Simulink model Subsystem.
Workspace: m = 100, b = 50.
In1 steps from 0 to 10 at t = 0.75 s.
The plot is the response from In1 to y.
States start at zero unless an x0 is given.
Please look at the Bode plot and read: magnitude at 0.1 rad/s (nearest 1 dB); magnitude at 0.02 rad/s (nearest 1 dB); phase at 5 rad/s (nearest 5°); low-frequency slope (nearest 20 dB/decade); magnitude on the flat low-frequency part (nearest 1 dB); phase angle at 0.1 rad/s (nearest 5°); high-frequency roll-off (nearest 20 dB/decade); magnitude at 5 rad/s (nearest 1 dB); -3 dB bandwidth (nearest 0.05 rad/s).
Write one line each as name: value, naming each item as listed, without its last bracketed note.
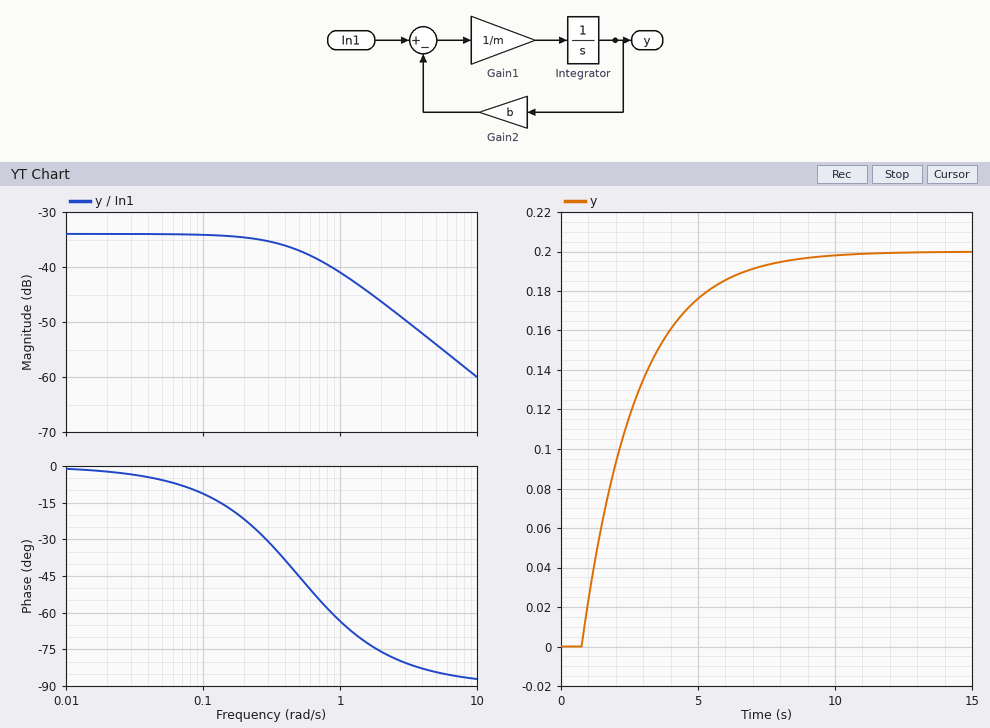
magnitude at 0.1 rad/s: -34 dB
magnitude at 0.02 rad/s: -34 dB
phase at 5 rad/s: -85°
low-frequency slope: 0 dB/decade
magnitude on the flat low-frequency part: -34 dB
phase angle at 0.1 rad/s: -10°
high-frequency roll-off: -20 dB/decade
magnitude at 5 rad/s: -54 dB
-3 dB bandwidth: 0.50 rad/s
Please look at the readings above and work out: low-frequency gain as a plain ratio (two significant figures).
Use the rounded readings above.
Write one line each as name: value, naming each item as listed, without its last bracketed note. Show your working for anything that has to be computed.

low-frequency gain as a plain ratio: 10^(-34 / 20) = 0.020
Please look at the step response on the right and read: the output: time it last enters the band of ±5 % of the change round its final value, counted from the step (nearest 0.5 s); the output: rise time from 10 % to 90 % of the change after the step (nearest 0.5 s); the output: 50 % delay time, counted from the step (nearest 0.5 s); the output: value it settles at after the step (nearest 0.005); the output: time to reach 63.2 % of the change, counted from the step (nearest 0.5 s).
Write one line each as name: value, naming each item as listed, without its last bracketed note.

the output: time it last enters the band of ±5 % of the change round its final value, counted from the step: 6.0 s
the output: rise time from 10 % to 90 % of the change after the step: 4.5 s
the output: 50 % delay time, counted from the step: 1.5 s
the output: value it settles at after the step: 0.200
the output: time to reach 63.2 % of the change, counted from the step: 2.0 s
